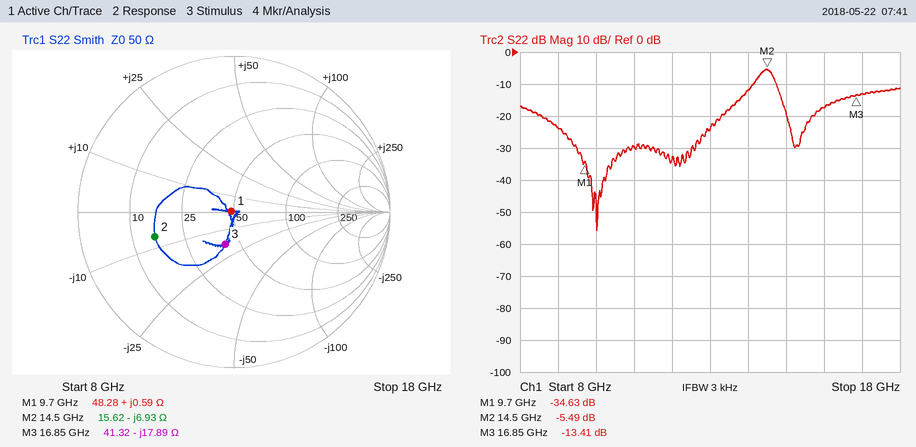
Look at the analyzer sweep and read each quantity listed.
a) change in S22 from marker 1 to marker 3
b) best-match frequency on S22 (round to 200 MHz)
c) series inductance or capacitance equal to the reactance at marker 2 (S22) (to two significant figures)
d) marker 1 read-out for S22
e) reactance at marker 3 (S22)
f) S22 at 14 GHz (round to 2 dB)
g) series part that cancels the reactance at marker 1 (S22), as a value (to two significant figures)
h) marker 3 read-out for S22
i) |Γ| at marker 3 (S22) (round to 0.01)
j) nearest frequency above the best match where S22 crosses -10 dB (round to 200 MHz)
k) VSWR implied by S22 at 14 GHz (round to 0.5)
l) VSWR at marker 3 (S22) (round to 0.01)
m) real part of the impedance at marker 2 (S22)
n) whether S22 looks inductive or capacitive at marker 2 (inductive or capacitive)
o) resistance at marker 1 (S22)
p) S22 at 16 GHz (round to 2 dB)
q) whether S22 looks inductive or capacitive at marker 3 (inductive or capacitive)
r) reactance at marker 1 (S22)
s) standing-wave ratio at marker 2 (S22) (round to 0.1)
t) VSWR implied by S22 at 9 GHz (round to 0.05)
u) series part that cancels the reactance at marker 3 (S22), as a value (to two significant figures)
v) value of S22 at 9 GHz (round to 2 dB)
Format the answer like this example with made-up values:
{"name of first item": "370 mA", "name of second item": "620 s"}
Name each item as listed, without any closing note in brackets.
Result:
{"change in S22 from marker 1 to marker 3": "21.22 dB", "best-match frequency on S22": "10.0 GHz", "series inductance or capacitance equal to the reactance at marker 2 (S22)": "1.6 pF", "marker 1 read-out for S22": "-34.63 dB", "reactance at marker 3": "-17.89 Ω", "S22 at 14 GHz": "-12 dB", "series part that cancels the reactance at marker 1 (S22), as a value": "28 pF", "marker 3 read-out for S22": "-13.41 dB", "|Γ| at marker 3 (S22)": "0.21", "nearest frequency above the best match where S22 crosses -10 dB": "14.2 GHz", "VSWR implied by S22 at 14 GHz": "1.5", "VSWR at marker 3 (S22)": "1.54", "real part of the impedance at marker 2": "15.62 Ω", "whether S22 looks inductive or capacitive at marker 2": "capacitive", "resistance at marker 1": "48.28 Ω", "S22 at 16 GHz": "-18 dB", "whether S22 looks inductive or capacitive at marker 3": "capacitive", "reactance at marker 1": "+0.59 Ω", "standing-wave ratio at marker 2 (S22)": "3.3", "VSWR implied by S22 at 9 GHz": "1.15", "series part that cancels the reactance at marker 3 (S22), as a value": "170 pH", "value of S22 at 9 GHz": "-24 dB"}
